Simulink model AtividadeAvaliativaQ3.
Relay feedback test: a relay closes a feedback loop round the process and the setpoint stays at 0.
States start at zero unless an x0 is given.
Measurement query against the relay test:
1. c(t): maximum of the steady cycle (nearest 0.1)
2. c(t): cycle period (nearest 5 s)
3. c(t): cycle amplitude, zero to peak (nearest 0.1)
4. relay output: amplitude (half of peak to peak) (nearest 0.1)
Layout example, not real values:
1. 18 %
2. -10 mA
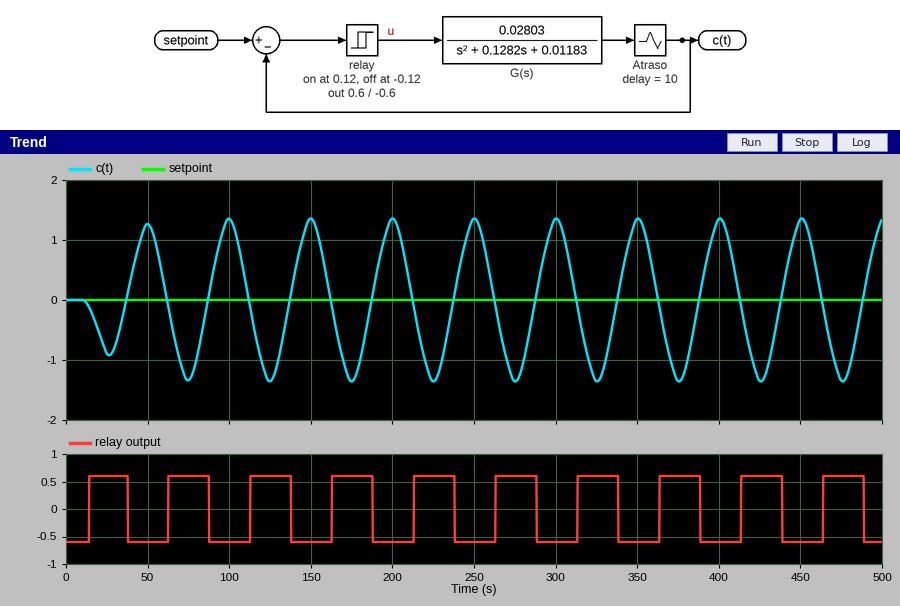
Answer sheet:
1. 1.4
2. 50 s
3. 1.4
4. 0.6
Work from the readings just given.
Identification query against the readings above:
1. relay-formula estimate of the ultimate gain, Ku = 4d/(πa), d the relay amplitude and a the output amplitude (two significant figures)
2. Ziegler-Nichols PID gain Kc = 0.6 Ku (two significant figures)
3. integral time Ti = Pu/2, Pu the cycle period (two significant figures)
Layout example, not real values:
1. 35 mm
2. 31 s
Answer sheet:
1. 0.55
2. 0.33
3. 25 s
